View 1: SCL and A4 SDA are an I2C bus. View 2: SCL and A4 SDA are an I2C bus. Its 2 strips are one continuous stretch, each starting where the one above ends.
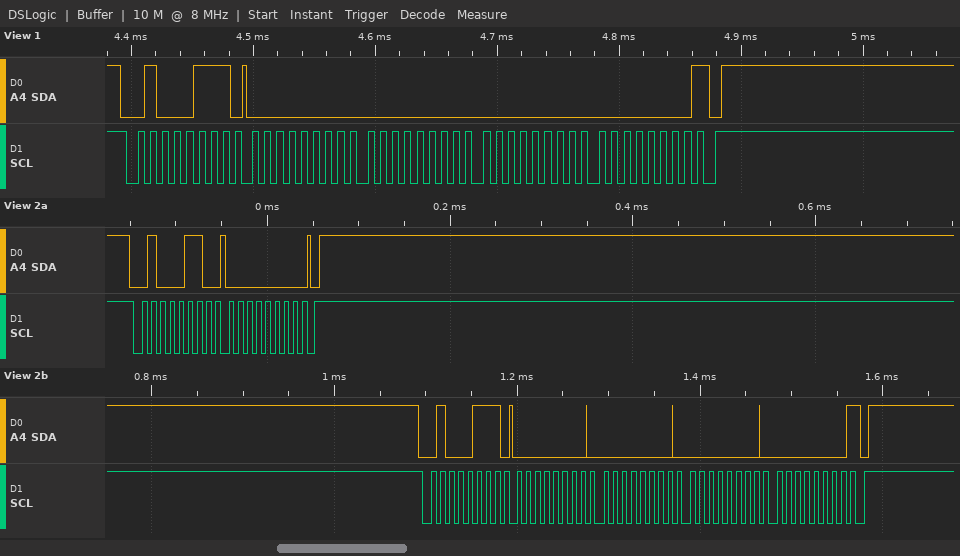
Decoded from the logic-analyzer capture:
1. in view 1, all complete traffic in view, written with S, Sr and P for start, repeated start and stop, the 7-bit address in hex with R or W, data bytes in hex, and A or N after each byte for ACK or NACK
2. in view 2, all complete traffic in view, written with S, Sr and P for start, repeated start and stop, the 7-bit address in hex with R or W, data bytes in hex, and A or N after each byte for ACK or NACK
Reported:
S 23R A 00 A 00 A 00 A 00 N P
S 23W A 00 A P S 23R A 00 A 00 A 00 A 00 N P
